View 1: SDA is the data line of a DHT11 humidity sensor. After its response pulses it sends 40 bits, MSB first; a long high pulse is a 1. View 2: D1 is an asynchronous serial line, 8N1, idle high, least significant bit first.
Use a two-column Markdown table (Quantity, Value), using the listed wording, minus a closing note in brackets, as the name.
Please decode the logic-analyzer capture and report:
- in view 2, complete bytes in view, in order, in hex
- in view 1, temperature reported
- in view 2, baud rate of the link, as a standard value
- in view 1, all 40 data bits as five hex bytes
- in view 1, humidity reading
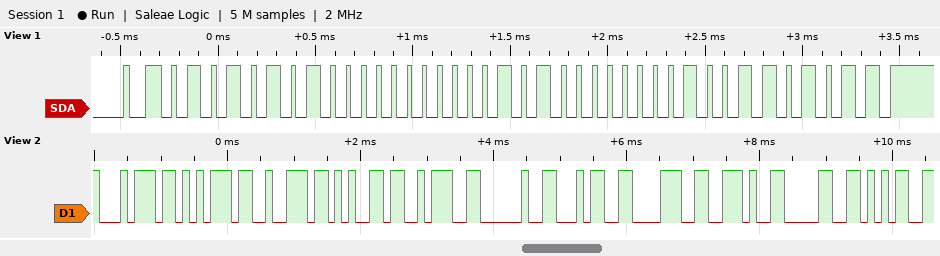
| Quantity | Value |
|---|---|
| in view 2, complete bytes in view, in order, in hex | 74 75 72 65 3A 20 34 38 2E 30 35 |
| in view 1, temperature reported | 20.2 °C |
| in view 2, baud rate of the link, as a standard value | 9600 baud |
| in view 1, all 40 data bits as five hex bytes | 55 00 14 02 6B |
| in view 1, humidity reading | 85 % |
